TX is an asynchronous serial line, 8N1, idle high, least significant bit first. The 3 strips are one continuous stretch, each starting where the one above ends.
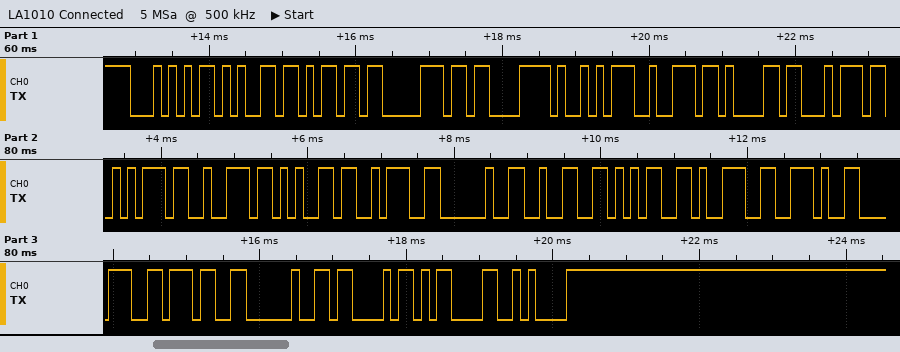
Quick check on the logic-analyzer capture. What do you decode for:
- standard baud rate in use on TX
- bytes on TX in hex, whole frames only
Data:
9600 baud
54 65 6D 70 C3 A9 72 61 74 75 72 65 3A 20 32 35 39 2E 38 37 20 43 0D 0A
